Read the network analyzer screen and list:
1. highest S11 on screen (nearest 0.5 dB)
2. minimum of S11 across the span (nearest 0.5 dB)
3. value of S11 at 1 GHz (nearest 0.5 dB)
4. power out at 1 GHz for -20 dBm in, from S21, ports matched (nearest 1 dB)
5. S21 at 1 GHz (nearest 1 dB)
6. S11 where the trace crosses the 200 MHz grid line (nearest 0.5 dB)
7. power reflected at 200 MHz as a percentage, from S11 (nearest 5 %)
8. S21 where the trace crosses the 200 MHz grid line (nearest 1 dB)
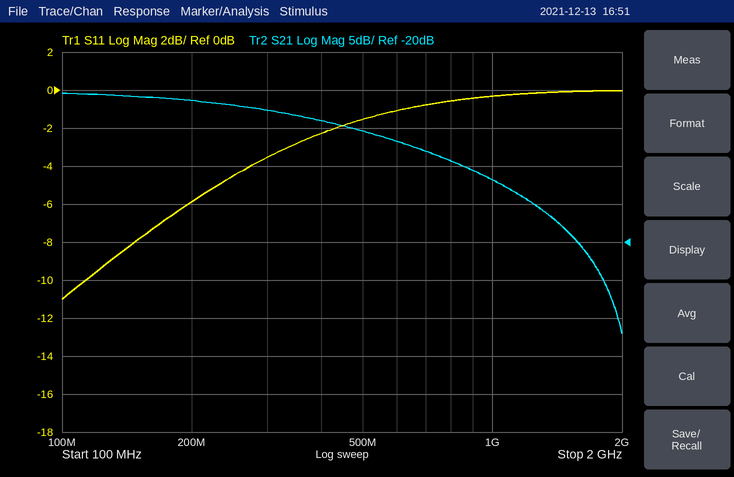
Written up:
0.0 dB
-11.0 dB
-0.5 dB
-32 dBm
-12 dB
-6.0 dB
25 %
-1 dB
